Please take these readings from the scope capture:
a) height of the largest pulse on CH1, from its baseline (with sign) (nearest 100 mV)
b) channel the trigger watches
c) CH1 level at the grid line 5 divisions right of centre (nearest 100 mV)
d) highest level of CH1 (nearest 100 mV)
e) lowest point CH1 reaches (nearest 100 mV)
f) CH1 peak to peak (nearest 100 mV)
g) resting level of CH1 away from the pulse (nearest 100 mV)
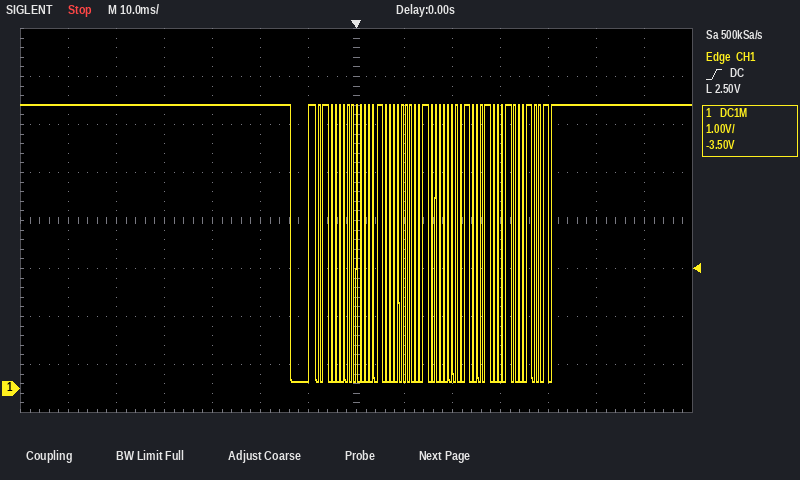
-5.8 V
CH1
5.9 V
5.9 V
100 mV
5.8 V
5.9 V
